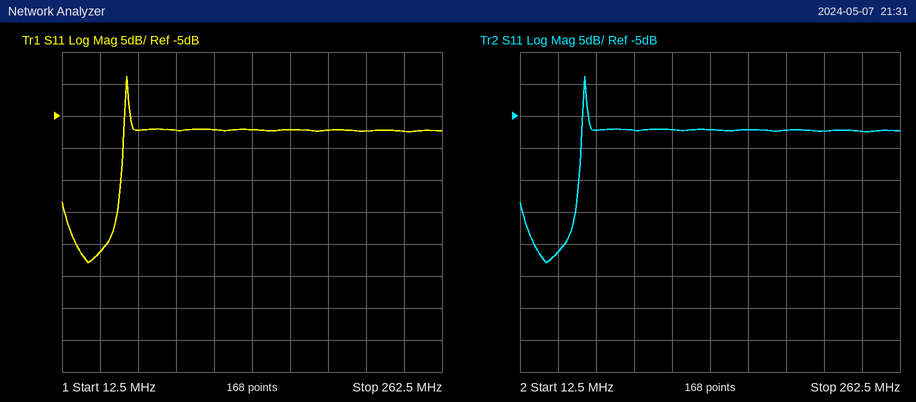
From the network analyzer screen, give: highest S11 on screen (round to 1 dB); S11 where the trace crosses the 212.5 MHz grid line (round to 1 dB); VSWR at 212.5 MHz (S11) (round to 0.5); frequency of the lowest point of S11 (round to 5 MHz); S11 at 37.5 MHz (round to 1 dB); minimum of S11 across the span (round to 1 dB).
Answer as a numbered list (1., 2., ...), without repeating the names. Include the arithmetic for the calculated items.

1. 1 dB
2. -7 dB
3. |Γ| = 10^(-7/20) = 0.4467; VSWR = (1 + 0.4467)/(1 − 0.4467) ≈ 2.61, so 2.5 to the nearest 0.5
4. 30 MHz
5. -26 dB
6. -28 dB
